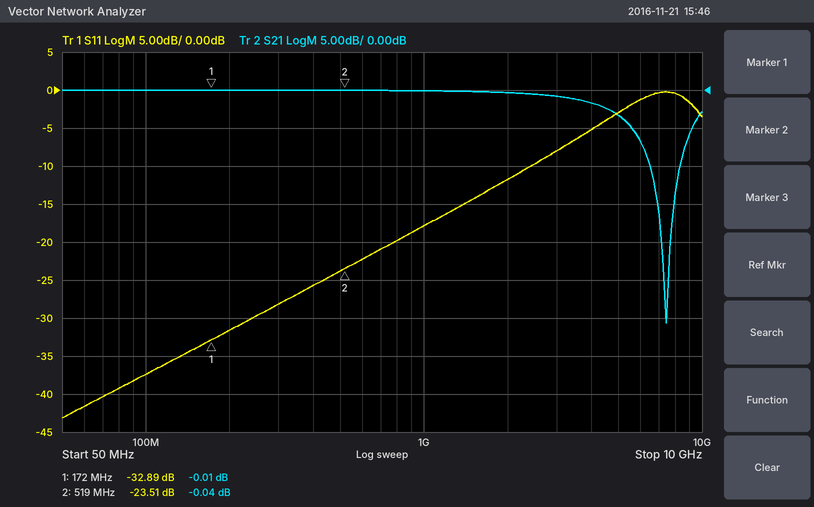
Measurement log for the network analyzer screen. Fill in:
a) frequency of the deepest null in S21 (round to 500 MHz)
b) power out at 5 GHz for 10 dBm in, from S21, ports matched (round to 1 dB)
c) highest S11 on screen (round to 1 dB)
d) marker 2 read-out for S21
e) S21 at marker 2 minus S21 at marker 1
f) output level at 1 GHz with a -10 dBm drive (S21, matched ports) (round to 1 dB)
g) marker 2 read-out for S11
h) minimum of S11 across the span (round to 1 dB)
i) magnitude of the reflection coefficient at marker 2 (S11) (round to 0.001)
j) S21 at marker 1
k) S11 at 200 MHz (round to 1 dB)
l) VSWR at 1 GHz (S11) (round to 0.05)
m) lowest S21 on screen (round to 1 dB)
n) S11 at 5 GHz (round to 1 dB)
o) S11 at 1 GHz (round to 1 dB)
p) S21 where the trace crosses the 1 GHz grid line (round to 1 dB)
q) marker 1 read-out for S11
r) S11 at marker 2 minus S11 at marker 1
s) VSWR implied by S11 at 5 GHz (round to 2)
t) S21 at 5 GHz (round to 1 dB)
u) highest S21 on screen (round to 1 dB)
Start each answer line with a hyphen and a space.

- 7.5 GHz
- 7 dBm
- 0 dB
- -0.04 dB
- -0.03 dB
- -10 dBm
- -23.51 dB
- -43 dB
- 0.067
- -0.01 dB
- -32 dB
- 1.30
- -31 dB
- -3 dB
- -18 dB
- 0 dB
- -32.89 dB
- 9.38 dB
- 6
- -3 dB
- 0 dB
